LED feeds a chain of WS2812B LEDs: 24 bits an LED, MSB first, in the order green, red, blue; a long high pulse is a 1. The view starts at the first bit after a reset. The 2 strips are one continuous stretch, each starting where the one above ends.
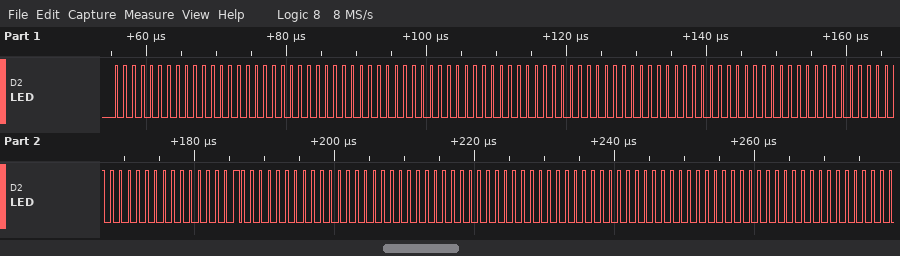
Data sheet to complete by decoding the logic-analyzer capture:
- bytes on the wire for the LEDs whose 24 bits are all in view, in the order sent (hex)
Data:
00 00 00 00 00 00 00 00 00 00 00 00 00 80 00 00 00 00 00 00 00
